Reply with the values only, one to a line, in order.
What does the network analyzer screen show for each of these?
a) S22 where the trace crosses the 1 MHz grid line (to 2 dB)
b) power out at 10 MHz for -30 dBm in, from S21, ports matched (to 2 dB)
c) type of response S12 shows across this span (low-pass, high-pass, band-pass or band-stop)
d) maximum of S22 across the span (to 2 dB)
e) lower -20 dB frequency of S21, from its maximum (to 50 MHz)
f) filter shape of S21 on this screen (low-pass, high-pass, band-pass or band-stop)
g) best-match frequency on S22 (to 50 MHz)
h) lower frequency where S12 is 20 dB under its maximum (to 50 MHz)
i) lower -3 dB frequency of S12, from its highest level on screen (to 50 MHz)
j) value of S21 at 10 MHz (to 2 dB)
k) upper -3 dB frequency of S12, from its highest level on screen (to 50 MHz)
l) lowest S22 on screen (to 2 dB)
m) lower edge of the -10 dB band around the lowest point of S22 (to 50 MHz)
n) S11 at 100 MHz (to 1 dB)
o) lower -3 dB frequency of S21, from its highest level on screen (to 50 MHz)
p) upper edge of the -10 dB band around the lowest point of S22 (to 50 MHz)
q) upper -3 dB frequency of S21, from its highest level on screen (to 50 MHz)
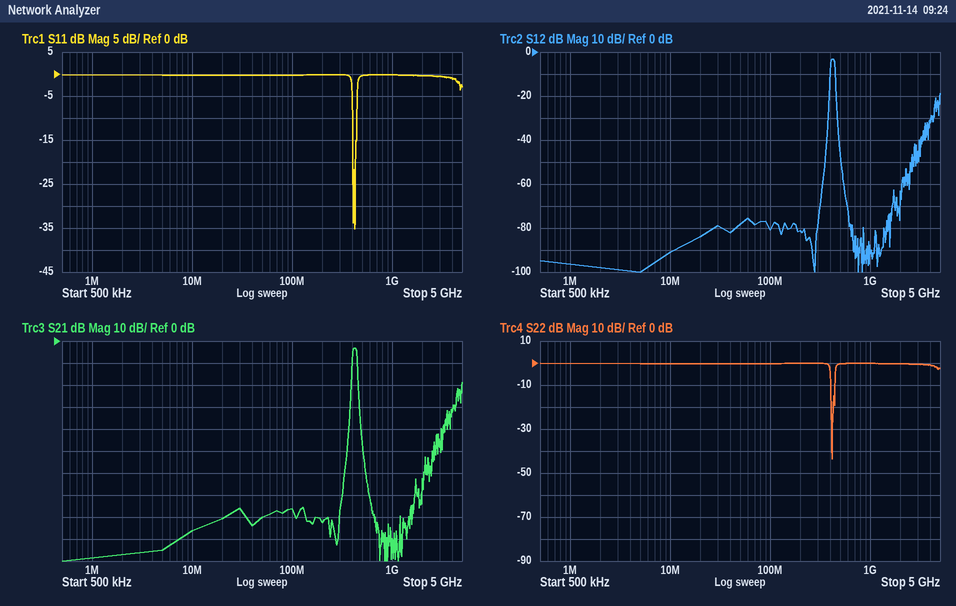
0 dB
-116 dBm
band-pass
0 dB
400 MHz
band-pass
400 MHz
400 MHz
400 MHz
-86 dB
450 MHz
-44 dB
400 MHz
0 dB
400 MHz
450 MHz
450 MHz
